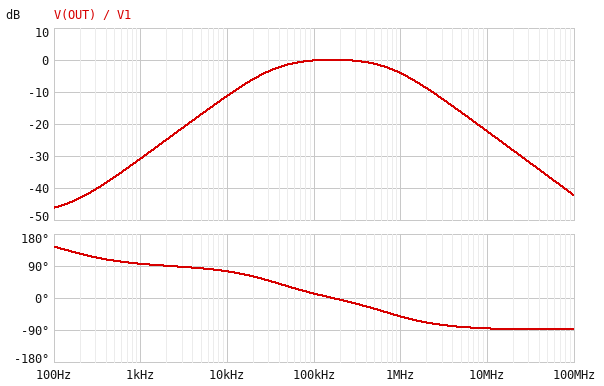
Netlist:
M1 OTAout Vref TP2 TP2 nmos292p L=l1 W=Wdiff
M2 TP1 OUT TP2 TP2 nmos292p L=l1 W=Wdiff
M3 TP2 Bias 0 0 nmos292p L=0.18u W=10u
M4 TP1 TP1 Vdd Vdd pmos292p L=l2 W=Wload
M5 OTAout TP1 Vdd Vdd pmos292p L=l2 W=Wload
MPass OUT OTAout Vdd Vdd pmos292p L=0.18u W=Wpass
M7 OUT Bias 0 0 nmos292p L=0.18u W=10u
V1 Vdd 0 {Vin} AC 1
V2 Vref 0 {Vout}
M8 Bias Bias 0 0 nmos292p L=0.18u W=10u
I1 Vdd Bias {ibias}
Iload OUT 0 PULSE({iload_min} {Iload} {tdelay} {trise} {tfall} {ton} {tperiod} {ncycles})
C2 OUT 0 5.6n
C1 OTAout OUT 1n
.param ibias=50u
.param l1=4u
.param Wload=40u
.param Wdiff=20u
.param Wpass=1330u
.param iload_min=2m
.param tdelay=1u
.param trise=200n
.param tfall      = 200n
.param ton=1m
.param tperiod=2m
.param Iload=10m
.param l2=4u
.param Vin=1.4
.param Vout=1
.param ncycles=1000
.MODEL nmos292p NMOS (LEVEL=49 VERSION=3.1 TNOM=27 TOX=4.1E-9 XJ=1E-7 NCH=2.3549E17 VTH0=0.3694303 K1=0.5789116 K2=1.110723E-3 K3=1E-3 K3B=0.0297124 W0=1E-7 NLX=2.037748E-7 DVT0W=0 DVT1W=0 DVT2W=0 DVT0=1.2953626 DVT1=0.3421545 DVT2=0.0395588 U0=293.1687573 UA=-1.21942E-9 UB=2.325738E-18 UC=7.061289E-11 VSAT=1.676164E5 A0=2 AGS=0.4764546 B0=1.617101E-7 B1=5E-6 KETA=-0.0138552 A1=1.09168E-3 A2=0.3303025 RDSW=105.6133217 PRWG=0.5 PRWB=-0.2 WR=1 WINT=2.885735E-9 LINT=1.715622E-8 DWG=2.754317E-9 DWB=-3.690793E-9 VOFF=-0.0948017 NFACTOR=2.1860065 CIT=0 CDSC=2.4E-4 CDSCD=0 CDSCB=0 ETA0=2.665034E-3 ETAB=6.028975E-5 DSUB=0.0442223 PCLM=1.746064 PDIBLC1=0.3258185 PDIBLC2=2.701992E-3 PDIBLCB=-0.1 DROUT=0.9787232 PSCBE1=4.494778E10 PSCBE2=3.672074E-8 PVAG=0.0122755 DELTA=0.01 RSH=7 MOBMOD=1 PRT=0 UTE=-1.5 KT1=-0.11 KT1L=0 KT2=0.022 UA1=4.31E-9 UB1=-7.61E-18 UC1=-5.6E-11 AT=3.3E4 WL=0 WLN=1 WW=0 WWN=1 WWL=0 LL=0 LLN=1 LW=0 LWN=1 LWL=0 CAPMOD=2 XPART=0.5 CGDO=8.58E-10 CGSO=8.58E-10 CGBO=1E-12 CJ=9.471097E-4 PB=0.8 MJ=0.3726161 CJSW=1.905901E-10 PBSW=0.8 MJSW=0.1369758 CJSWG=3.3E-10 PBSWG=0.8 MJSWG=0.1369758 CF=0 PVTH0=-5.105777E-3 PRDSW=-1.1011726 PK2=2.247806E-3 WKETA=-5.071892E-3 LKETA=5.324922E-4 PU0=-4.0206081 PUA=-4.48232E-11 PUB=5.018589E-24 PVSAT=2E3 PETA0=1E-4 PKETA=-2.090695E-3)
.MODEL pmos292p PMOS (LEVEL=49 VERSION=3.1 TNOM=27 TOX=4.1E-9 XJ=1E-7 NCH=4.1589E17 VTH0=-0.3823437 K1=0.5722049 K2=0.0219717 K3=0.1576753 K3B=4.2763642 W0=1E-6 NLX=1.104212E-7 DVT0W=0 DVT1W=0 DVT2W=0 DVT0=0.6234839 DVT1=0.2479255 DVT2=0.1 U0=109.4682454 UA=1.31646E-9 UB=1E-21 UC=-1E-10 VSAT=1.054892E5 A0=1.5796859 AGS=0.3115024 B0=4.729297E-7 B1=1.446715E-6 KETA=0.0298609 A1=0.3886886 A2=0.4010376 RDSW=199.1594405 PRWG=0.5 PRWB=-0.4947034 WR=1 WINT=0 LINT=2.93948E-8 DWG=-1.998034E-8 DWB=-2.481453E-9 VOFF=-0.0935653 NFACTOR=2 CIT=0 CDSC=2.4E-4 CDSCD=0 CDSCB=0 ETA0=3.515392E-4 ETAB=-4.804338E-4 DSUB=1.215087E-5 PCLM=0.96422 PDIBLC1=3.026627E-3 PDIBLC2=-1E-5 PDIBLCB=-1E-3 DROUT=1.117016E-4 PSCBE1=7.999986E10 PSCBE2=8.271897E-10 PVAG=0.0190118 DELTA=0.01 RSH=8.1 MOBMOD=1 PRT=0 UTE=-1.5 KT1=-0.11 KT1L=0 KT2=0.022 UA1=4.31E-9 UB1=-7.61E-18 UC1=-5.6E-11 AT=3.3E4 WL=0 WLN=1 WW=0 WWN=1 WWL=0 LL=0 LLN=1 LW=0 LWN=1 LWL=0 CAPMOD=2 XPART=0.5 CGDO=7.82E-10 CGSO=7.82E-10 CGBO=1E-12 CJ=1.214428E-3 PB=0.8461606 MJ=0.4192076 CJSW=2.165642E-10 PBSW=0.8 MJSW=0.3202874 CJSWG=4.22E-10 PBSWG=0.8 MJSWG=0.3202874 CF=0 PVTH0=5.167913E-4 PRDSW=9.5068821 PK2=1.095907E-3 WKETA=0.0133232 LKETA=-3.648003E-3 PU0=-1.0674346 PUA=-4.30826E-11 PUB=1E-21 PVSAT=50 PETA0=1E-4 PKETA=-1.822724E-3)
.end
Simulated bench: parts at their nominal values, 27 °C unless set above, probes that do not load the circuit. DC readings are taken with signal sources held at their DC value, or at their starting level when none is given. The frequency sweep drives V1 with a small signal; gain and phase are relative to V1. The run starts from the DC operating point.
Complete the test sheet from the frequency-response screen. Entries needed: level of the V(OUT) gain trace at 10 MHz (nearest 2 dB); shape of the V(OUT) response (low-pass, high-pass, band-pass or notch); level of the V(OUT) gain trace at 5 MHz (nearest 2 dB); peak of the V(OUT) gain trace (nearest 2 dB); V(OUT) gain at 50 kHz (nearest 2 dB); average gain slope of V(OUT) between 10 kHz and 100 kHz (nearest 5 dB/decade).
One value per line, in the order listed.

-22 dB
band-pass
-16 dB
0 dB
-2 dB
10 dB/decade
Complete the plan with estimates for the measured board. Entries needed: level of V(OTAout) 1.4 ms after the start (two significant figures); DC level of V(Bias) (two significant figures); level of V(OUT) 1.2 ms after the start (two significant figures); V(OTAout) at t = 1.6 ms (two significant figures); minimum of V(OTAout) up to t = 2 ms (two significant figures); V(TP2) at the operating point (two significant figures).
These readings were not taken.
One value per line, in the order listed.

840 mV
540 mV
1.0 V
840 mV
640 mV
410 mV
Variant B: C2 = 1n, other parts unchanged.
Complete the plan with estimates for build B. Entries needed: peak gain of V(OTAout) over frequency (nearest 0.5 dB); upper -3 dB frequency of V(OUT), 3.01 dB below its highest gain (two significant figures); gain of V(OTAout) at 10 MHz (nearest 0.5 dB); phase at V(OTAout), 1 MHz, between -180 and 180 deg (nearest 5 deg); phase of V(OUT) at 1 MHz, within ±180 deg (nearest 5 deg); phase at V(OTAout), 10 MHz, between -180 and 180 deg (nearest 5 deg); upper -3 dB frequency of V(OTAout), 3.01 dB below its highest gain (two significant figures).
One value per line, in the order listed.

0 dB
4.3 MHz
-8.0 dB
-15 deg
-10 deg
-65 deg
4.2 MHz
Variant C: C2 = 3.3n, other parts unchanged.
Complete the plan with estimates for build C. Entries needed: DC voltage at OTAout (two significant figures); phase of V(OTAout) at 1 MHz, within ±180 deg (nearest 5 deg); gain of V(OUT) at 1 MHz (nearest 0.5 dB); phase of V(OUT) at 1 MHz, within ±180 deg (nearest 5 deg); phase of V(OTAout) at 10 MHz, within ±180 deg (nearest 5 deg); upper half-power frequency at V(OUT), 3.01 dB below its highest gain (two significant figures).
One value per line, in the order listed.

840 mV
-40 deg
-2.0 dB
-35 deg
-80 deg
1.3 MHz
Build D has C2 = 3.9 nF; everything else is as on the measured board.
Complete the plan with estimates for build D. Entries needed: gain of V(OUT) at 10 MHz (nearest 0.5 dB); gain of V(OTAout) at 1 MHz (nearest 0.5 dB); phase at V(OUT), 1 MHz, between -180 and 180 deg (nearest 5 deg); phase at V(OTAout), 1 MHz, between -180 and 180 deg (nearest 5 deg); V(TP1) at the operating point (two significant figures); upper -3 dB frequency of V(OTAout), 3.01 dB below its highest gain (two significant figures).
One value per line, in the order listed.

-19.0 dB
-2.5 dB
-40 deg
-45 deg
720 mV
1.1 MHz
